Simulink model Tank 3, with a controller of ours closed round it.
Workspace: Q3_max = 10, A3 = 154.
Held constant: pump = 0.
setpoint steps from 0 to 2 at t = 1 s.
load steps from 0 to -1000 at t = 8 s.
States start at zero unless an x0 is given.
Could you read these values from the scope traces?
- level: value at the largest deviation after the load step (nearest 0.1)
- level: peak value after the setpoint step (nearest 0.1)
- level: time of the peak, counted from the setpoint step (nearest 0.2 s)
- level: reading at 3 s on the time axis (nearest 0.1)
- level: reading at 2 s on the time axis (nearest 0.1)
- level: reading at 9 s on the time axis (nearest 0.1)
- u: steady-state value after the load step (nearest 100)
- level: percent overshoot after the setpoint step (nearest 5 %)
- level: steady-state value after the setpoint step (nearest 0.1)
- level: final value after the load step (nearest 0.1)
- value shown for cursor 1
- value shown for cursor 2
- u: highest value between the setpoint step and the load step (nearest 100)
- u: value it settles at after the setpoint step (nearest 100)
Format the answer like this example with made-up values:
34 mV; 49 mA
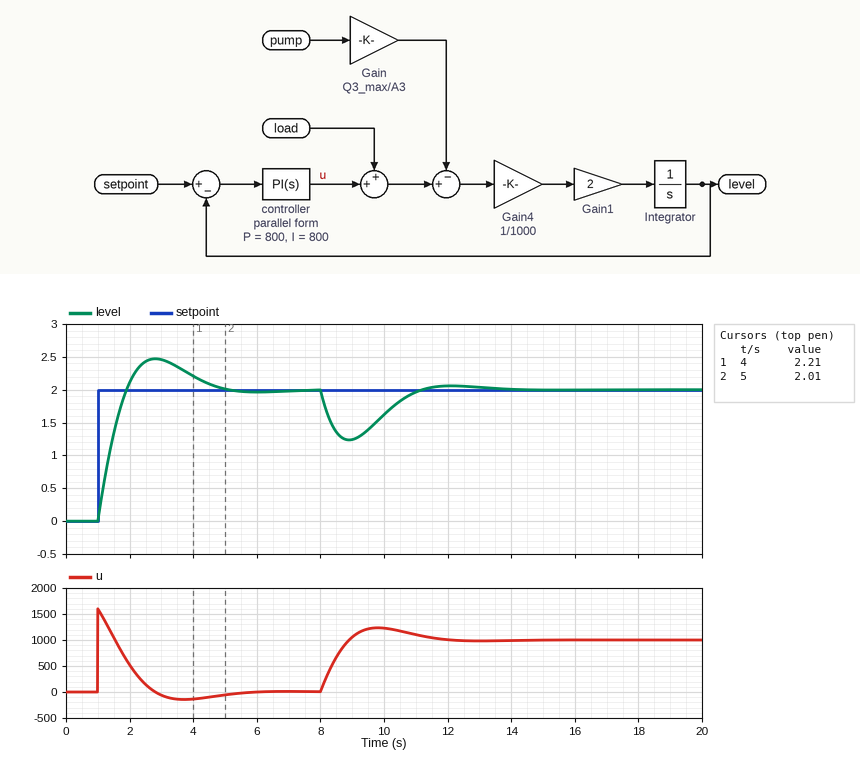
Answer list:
1.2; 2.5; 1.8 s; 2.5; 2.1; 1.2; 1000; 25 %; 2.0; 2.0; 2.21; 2.01; 1600; 0
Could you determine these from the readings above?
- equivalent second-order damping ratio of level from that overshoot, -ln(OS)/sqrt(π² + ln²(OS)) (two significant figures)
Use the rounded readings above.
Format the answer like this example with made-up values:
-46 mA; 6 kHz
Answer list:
0.40
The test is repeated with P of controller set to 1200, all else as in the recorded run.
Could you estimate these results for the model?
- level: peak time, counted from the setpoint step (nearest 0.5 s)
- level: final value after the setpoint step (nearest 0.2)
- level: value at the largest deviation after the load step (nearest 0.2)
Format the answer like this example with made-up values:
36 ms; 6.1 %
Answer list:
1.5 s; 2.0; 1.4
